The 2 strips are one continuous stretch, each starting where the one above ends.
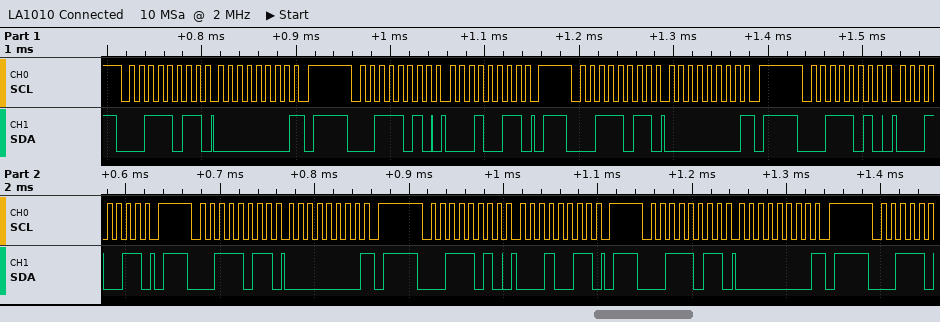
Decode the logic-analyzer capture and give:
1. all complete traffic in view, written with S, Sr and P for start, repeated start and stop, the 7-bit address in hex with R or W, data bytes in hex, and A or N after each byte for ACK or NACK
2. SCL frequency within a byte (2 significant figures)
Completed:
S 1DR A 00 N P S 1DW A 13 A P S 1DR A 00 N P S 1DW A 13 A P S 1DR A 00 N P S 1DW A 13 A P S 1DR A 00 N P
100 kHz
